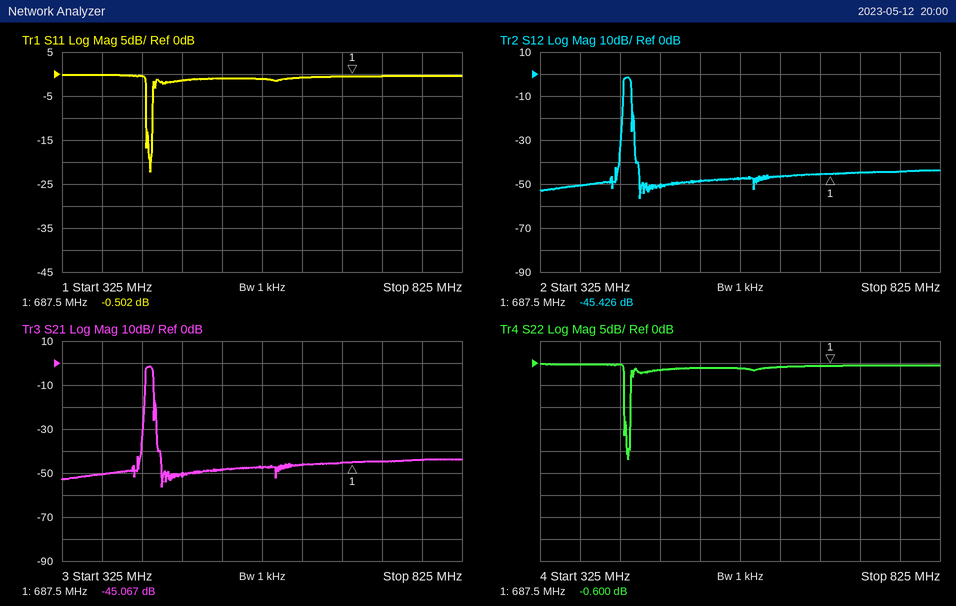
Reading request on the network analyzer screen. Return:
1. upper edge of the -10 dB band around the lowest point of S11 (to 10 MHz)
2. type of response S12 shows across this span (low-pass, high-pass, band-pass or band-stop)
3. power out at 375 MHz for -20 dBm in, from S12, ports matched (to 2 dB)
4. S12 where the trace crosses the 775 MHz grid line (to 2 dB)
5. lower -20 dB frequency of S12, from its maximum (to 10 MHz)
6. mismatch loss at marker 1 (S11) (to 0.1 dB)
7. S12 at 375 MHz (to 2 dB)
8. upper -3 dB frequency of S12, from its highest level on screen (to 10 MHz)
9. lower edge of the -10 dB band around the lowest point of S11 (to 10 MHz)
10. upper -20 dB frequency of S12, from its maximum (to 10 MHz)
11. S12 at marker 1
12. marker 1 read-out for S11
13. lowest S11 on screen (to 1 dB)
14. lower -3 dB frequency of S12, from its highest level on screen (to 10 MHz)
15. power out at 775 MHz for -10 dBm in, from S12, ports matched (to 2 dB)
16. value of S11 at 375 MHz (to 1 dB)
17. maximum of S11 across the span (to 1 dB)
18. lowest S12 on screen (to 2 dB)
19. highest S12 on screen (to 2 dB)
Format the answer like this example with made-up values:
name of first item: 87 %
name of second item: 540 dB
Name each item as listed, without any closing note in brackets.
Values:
upper edge of the -10 dB band around the lowest point of S11: 440 MHz
type of response S12 shows across this span: band-pass
power out at 375 MHz for -20 dBm in, from S12, ports matched: -70 dBm
S12 where the trace crosses the 775 MHz grid line: -44 dB
lower -20 dB frequency of S12, from its maximum: 430 MHz
mismatch loss at marker 1 (S11): 9.6 dB
S12 at 375 MHz: -50 dB
upper -3 dB frequency of S12, from its highest level on screen: 440 MHz
lower edge of the -10 dB band around the lowest point of S11: 430 MHz
upper -20 dB frequency of S12, from its maximum: 440 MHz
S12 at marker 1: -45.426 dB
marker 1 read-out for S11: -0.502 dB
lowest S11 on screen: -22 dB
lower -3 dB frequency of S12, from its highest level on screen: 430 MHz
power out at 775 MHz for -10 dBm in, from S12, ports matched: -54 dBm
value of S11 at 375 MHz: 0 dB
maximum of S11 across the span: 0 dB
lowest S12 on screen: -56 dB
highest S12 on screen: -2 dB
